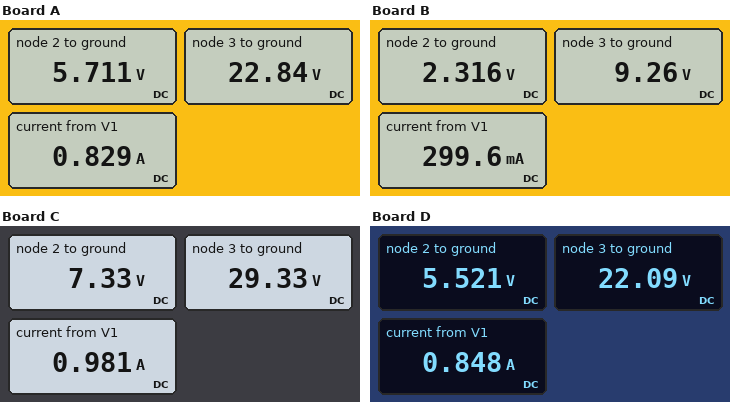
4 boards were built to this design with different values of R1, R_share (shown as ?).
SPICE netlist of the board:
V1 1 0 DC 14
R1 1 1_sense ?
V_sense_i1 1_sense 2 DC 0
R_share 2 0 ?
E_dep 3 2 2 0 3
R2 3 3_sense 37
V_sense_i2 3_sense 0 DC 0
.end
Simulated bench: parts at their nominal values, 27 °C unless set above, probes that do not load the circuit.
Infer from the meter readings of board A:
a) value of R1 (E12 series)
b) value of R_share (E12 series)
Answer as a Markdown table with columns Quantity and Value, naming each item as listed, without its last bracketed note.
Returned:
| Quantity | Value |
|---|---|
| value of R1 | 10 Ω |
| value of R_share | 27 Ω |
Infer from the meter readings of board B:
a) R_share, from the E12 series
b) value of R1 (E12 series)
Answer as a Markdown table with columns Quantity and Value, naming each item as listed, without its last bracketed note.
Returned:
| Quantity | Value |
|---|---|
| R_share, from the E12 series | 47 Ω |
| value of R1 | 39 Ω |
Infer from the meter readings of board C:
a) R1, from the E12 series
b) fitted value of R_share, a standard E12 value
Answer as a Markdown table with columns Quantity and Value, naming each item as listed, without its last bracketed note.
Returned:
| Quantity | Value |
|---|---|
| R1, from the E12 series | 6.8 Ω |
| fitted value of R_share, a standard E12 value | 39 Ω |
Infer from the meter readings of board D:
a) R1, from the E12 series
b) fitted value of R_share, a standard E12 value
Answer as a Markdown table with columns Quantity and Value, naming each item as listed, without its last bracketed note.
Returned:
| Quantity | Value |
|---|---|
| R1, from the E12 series | 10 Ω |
| fitted value of R_share, a standard E12 value | 22 Ω |
